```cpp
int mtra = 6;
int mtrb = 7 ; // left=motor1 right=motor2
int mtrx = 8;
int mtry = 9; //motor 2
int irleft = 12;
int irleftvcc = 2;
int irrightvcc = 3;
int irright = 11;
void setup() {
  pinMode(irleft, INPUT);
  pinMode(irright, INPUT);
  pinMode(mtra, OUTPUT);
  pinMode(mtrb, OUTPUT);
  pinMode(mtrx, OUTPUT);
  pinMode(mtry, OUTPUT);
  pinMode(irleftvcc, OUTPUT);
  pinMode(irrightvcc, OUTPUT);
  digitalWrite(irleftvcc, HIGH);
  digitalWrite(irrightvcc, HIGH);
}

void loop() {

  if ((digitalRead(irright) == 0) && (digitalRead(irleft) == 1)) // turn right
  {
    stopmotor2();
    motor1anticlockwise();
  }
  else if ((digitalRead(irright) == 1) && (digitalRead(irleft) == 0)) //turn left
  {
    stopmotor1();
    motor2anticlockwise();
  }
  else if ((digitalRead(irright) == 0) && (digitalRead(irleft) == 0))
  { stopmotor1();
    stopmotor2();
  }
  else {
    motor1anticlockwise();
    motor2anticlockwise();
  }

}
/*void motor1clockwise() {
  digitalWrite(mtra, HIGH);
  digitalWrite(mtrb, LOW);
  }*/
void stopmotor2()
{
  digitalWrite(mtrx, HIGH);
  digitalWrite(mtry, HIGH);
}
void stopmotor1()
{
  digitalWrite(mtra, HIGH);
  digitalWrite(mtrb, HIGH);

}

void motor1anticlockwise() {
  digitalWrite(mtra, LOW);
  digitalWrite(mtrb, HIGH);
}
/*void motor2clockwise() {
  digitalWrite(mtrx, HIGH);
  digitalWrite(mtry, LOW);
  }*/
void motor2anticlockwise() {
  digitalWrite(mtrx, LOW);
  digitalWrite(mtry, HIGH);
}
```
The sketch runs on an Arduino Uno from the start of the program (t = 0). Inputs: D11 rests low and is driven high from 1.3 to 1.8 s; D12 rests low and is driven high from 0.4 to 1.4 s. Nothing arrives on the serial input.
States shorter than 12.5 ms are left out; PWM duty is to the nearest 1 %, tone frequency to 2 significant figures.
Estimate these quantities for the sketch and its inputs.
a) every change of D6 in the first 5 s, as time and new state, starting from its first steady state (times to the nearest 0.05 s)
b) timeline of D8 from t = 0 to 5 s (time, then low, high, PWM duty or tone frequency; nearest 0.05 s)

0 s high; 0.4 s low; 1.4 s high
0 s high; 1.3 s low; 1.8 s high
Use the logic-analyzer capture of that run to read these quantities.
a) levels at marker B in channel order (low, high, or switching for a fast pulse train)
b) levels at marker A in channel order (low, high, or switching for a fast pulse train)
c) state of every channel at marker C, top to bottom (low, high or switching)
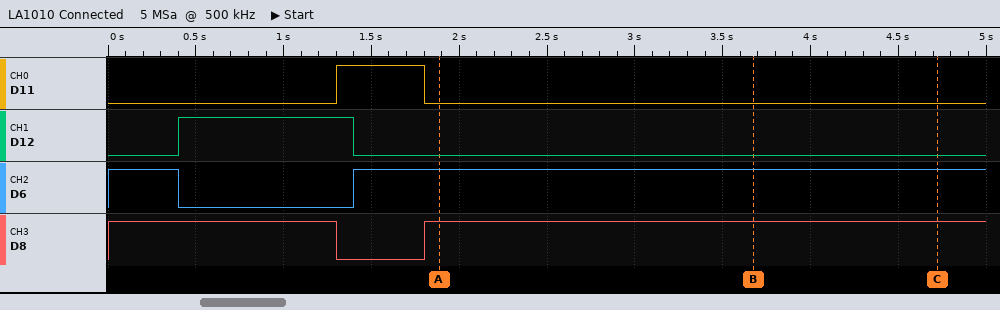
D11 low, D12 low, D6 high, D8 high
D11 low, D12 low, D6 high, D8 high
D11 low, D12 low, D6 high, D8 high
